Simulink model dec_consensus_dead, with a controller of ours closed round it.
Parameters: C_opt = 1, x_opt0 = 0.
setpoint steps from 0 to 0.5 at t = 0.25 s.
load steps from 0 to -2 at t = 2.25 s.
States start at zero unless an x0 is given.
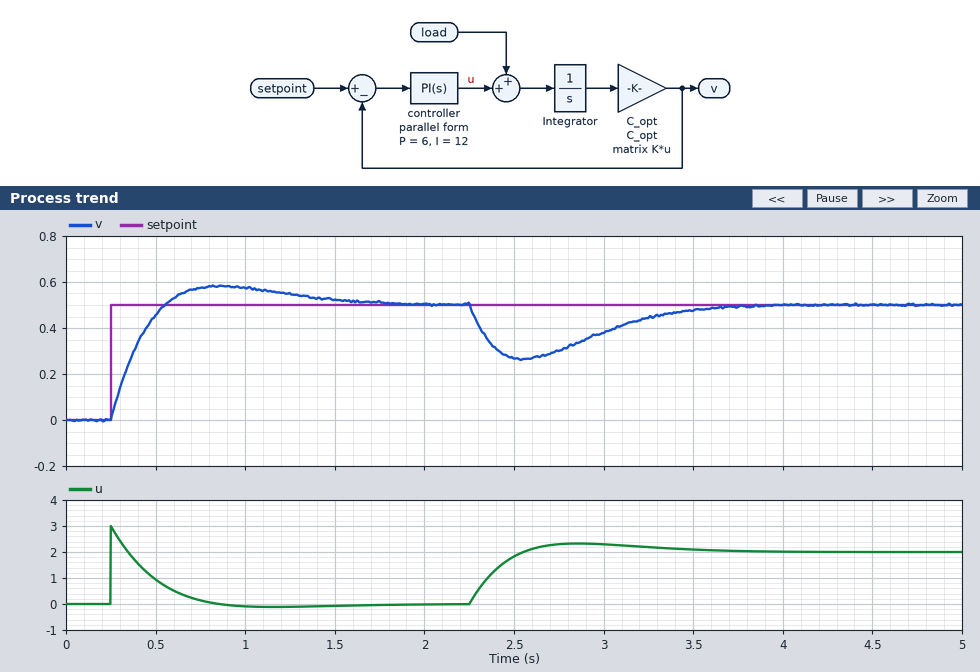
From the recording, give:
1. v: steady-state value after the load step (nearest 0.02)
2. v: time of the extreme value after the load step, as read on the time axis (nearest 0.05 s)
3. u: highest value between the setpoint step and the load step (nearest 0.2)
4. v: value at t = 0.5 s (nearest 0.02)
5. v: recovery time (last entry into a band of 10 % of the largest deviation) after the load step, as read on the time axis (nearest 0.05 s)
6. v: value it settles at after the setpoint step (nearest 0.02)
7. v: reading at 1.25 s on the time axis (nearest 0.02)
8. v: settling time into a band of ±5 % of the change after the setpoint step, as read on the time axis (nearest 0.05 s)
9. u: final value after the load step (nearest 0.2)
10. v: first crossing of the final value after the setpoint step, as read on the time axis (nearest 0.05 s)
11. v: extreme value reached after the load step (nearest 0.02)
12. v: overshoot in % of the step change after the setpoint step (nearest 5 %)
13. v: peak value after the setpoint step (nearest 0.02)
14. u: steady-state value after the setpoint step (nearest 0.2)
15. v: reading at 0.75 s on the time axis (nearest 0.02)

0.50
2.55 s
3.0
0.46
3.50 s
0.50
0.54
1.50 s
2.0
0.55 s
0.26
15 %
0.58
0.0
0.58
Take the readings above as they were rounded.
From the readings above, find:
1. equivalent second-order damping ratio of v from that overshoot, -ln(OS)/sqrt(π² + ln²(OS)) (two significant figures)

0.52
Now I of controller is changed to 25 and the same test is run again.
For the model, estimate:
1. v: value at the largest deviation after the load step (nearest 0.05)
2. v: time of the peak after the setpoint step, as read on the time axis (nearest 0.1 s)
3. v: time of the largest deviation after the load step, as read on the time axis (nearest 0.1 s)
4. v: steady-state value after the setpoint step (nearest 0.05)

0.30
0.7 s
2.5 s
0.50
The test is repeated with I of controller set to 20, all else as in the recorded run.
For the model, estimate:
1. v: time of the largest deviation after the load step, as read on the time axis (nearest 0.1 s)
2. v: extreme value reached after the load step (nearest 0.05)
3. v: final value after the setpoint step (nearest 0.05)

2.5 s
0.30
0.50
